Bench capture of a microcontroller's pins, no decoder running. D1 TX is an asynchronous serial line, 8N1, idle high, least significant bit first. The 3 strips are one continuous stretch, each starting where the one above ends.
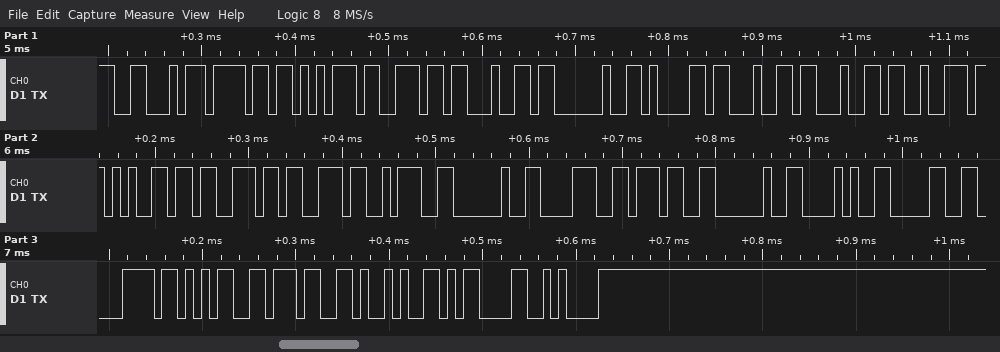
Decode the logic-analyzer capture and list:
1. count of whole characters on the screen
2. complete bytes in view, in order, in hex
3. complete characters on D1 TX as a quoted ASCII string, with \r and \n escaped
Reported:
26
46 6F 75 6E 64 20 61 64 64 72 65 73 73 3A 20 38 37 20 28 30 78 35 37 29 0D 0A
"Found address: 87 (0x57)\r\n"
